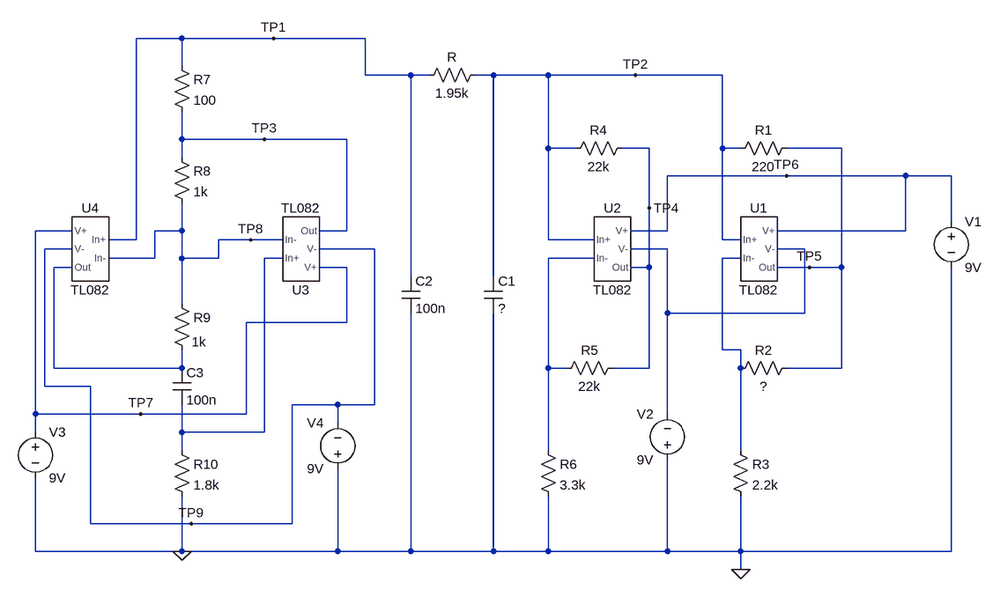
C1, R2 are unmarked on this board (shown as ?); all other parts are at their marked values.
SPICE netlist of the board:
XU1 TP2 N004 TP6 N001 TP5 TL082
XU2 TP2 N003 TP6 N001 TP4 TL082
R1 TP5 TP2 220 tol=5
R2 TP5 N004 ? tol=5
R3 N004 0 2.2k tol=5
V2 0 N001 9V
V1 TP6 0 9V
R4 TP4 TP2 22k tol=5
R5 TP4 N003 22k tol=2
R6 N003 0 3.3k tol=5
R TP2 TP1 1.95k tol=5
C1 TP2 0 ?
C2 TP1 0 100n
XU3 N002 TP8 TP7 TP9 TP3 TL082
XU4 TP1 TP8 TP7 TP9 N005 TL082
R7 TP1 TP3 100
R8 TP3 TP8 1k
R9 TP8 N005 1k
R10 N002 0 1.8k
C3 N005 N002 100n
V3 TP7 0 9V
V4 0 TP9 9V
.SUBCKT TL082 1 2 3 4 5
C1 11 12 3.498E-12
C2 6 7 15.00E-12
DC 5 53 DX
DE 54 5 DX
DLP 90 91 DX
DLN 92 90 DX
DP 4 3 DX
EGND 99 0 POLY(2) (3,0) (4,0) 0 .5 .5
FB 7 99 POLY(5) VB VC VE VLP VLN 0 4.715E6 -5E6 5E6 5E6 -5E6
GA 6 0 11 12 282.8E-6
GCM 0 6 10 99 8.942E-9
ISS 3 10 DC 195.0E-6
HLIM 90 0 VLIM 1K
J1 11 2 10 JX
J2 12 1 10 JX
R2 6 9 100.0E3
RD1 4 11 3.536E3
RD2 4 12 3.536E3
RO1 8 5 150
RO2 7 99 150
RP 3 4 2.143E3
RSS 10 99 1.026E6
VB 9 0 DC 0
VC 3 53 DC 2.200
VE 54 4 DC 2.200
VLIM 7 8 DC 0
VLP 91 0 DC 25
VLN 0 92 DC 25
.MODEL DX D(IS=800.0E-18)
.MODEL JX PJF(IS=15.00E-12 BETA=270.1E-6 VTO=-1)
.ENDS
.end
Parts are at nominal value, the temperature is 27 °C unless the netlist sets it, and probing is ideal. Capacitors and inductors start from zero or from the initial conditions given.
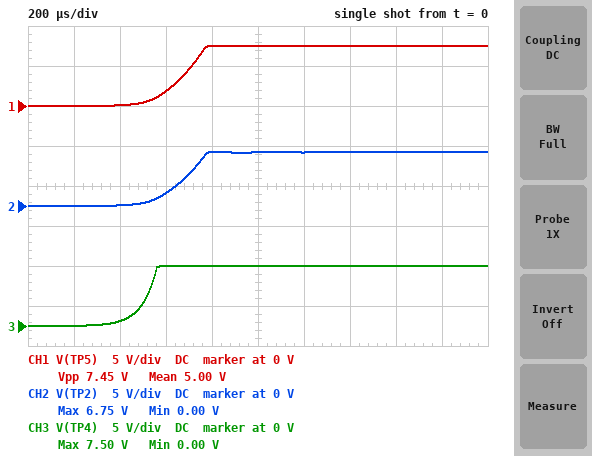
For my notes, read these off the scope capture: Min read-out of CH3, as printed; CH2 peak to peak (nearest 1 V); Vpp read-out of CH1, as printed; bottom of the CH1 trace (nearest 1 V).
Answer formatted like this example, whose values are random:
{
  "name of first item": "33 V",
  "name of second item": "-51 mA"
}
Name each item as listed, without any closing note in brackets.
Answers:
{
  "Min read-out of CH3, as printed": "0.00 V",
  "CH2 peak to peak": "7 V",
  "Vpp read-out of CH1, as printed": "7.45 V",
  "bottom of the CH1 trace": "0 V"
}
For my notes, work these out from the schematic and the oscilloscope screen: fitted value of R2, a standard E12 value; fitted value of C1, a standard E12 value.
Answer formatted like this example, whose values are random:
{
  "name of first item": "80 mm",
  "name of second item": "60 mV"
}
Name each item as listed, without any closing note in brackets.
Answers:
{
  "fitted value of R2, a standard E12 value": "330 Ω",
  "fitted value of C1, a standard E12 value": "33 nF"
}
